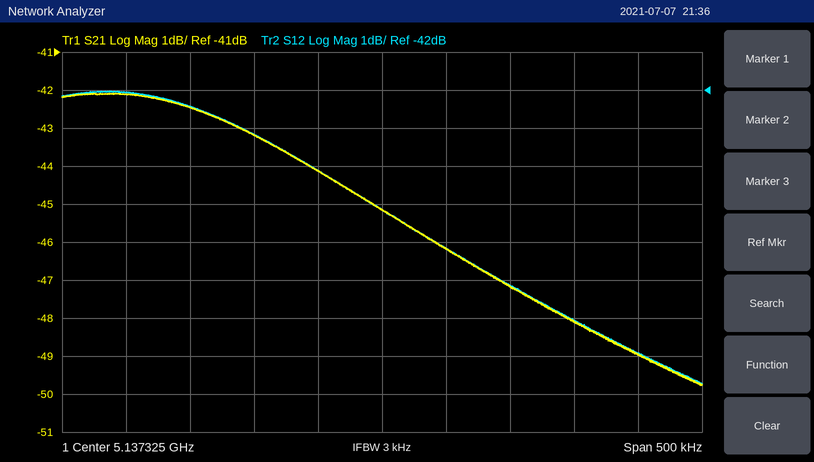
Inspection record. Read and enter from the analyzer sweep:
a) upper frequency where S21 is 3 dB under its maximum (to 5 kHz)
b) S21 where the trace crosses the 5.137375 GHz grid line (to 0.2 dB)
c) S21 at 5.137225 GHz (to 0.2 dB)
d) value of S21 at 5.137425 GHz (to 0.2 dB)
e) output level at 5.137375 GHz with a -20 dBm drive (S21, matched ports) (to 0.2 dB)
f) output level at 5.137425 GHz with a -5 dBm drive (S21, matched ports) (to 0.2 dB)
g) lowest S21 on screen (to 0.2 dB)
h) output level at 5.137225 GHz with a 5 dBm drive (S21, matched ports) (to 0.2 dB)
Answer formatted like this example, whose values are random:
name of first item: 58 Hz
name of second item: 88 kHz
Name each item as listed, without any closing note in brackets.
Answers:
upper frequency where S21 is 3 dB under its maximum: 5.137320 GHz
S21 where the trace crosses the 5.137375 GHz grid line: -46.2 dB
S21 at 5.137225 GHz: -43.2 dB
value of S21 at 5.137425 GHz: -47.2 dB
output level at 5.137375 GHz with a -20 dBm drive (S21, matched ports): -66.2 dBm
output level at 5.137425 GHz with a -5 dBm drive (S21, matched ports): -52.2 dBm
lowest S21 on screen: -49.8 dB
output level at 5.137225 GHz with a 5 dBm drive (S21, matched ports): -38.2 dBm
